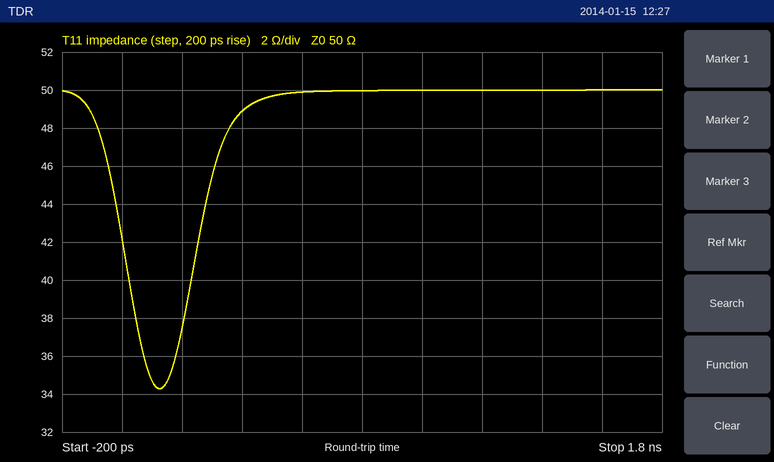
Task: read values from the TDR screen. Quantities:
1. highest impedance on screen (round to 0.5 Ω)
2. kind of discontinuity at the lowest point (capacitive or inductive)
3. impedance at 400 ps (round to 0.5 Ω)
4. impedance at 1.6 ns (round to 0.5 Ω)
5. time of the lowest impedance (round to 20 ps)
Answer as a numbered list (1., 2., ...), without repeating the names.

1. 50.0 Ω
2. capacitive
3. 49.0 Ω
4. 50.0 Ω
5. 120 ps
